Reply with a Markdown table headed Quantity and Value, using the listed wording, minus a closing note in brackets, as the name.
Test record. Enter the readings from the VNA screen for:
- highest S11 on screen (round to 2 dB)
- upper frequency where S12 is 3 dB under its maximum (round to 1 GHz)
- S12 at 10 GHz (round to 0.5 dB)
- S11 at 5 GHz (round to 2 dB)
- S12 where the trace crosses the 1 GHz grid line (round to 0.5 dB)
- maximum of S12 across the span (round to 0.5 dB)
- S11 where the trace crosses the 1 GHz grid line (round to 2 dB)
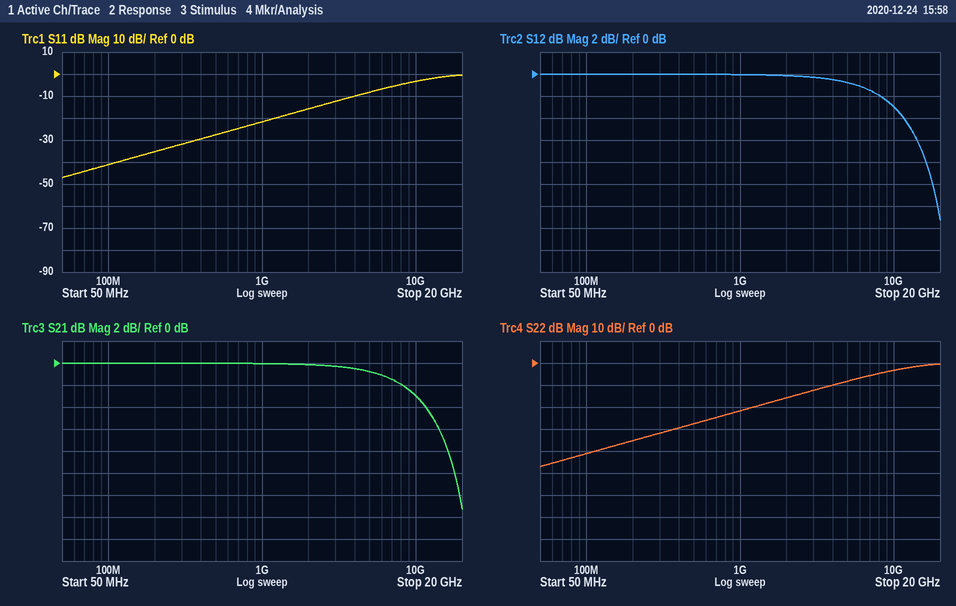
| Quantity | Value |
|---|---|
| highest S11 on screen | 0 dB |
| upper frequency where S12 is 3 dB under its maximum | 10 GHz |
| S12 at 10 GHz | -3.0 dB |
| S11 at 5 GHz | -8 dB |
| S12 where the trace crosses the 1 GHz grid line | 0.0 dB |
| maximum of S12 across the span | 0.0 dB |
| S11 where the trace crosses the 1 GHz grid line | -22 dB |
